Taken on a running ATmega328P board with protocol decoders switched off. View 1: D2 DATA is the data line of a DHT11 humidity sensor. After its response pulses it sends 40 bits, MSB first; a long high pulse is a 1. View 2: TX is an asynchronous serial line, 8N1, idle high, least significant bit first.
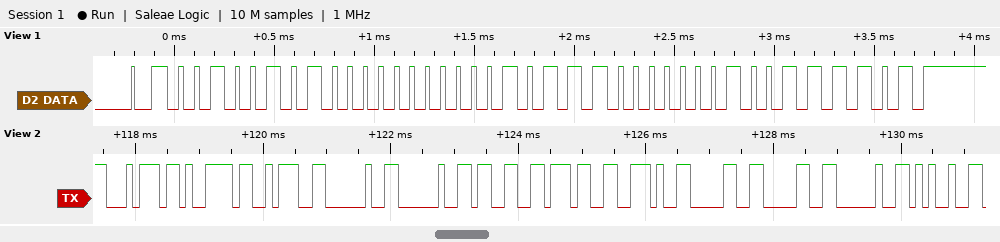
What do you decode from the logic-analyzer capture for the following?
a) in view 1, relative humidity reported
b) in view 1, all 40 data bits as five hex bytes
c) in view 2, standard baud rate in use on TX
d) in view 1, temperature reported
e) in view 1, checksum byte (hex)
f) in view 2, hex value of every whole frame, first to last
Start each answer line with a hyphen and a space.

- 37 %
- 25 00 17 01 3D
- 9600 baud
- 23.1 °C
- 0x3D
- 74 79 3A 20 20 33 37 2E 30 30 20 25
